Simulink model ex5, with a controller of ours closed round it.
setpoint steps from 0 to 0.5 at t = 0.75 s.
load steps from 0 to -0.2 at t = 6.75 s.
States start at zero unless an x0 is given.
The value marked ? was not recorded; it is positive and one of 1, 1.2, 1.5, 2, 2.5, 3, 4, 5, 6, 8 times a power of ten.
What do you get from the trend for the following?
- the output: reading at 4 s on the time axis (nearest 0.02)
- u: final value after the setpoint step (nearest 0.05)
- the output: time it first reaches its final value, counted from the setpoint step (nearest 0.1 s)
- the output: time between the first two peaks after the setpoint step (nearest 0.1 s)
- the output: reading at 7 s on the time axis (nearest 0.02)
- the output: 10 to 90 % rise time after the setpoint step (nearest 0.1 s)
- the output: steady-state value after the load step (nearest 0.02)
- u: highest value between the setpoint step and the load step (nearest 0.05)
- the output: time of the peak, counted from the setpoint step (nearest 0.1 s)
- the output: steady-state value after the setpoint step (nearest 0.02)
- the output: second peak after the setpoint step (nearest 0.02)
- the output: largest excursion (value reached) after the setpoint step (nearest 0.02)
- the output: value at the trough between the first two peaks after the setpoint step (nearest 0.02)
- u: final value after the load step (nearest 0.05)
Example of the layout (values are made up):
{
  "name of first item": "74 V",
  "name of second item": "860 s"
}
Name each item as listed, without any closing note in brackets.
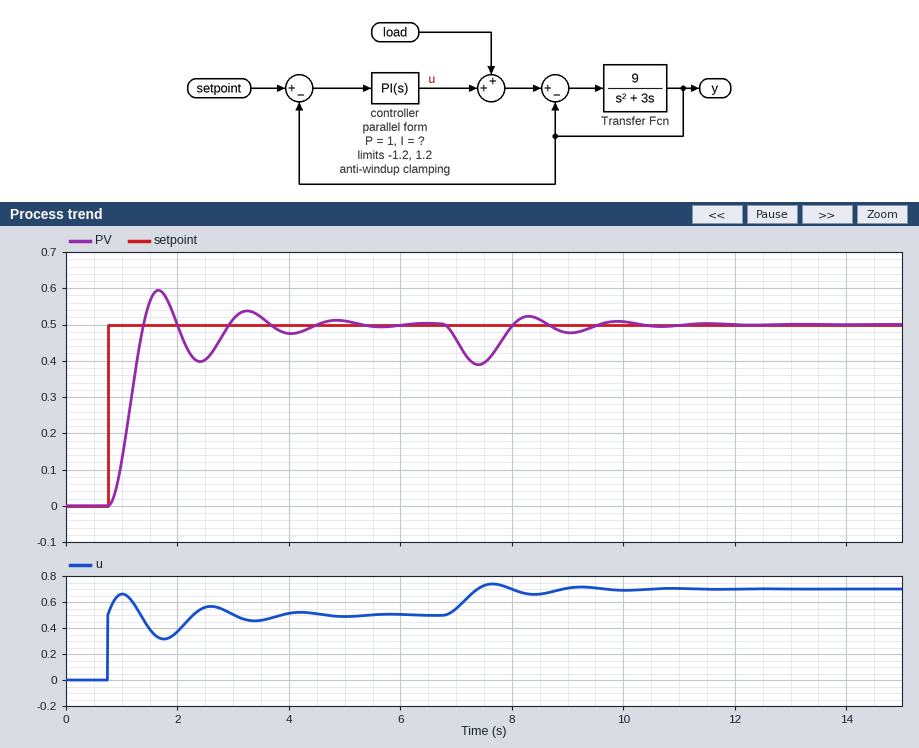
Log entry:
{
  "the output: reading at 4 s on the time axis": "0.48",
  "u: final value after the setpoint step": "0.50",
  "the output: time it first reaches its final value, counted from the setpoint step": "0.6 s",
  "the output: time between the first two peaks after the setpoint step": "1.6 s",
  "the output: reading at 7 s on the time axis": "0.46",
  "the output: 10 to 90 % rise time after the setpoint step": "0.4 s",
  "the output: steady-state value after the load step": "0.50",
  "u: highest value between the setpoint step and the load step": "0.65",
  "the output: time of the peak, counted from the setpoint step": "0.9 s",
  "the output: steady-state value after the setpoint step": "0.50",
  "the output: second peak after the setpoint step": "0.54",
  "the output: largest excursion (value reached) after the setpoint step": "0.60",
  "the output: value at the trough between the first two peaks after the setpoint step": "0.40",
  "u: final value after the load step": "0.70"
}
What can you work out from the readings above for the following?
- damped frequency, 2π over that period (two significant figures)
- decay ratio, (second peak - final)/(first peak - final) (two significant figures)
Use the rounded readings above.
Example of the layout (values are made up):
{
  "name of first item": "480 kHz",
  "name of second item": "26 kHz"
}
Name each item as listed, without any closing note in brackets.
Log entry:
{
  "damped frequency, 2π over that period": "3.9 rad/s",
  "decay ratio, (second peak - final)/(first peak - final)": "0.40"
}
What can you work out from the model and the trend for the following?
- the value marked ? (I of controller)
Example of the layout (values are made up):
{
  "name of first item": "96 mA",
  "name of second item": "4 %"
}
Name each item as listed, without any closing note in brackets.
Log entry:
{
  "the value marked ?": "2.5"
}
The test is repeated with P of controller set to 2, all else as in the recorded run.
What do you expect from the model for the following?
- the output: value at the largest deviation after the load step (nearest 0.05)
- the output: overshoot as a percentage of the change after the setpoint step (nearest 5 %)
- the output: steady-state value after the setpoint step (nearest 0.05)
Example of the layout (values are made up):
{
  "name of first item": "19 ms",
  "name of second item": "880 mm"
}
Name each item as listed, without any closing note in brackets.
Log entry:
{
  "the output: value at the largest deviation after the load step": "0.40",
  "the output: overshoot as a percentage of the change after the setpoint step": "20 %",
  "the output: steady-state value after the setpoint step": "0.50"
}
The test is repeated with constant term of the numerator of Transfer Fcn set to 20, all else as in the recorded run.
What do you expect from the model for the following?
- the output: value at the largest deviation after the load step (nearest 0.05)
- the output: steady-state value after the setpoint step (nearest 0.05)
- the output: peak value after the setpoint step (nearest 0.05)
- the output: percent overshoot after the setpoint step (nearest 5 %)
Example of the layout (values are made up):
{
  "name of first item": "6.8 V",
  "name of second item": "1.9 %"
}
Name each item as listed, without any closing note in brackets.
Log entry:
{
  "the output: value at the largest deviation after the load step": "0.35",
  "the output: steady-state value after the setpoint step": "0.50",
  "the output: peak value after the setpoint step": "0.55",
  "the output: percent overshoot after the setpoint step": "10 %"
}
